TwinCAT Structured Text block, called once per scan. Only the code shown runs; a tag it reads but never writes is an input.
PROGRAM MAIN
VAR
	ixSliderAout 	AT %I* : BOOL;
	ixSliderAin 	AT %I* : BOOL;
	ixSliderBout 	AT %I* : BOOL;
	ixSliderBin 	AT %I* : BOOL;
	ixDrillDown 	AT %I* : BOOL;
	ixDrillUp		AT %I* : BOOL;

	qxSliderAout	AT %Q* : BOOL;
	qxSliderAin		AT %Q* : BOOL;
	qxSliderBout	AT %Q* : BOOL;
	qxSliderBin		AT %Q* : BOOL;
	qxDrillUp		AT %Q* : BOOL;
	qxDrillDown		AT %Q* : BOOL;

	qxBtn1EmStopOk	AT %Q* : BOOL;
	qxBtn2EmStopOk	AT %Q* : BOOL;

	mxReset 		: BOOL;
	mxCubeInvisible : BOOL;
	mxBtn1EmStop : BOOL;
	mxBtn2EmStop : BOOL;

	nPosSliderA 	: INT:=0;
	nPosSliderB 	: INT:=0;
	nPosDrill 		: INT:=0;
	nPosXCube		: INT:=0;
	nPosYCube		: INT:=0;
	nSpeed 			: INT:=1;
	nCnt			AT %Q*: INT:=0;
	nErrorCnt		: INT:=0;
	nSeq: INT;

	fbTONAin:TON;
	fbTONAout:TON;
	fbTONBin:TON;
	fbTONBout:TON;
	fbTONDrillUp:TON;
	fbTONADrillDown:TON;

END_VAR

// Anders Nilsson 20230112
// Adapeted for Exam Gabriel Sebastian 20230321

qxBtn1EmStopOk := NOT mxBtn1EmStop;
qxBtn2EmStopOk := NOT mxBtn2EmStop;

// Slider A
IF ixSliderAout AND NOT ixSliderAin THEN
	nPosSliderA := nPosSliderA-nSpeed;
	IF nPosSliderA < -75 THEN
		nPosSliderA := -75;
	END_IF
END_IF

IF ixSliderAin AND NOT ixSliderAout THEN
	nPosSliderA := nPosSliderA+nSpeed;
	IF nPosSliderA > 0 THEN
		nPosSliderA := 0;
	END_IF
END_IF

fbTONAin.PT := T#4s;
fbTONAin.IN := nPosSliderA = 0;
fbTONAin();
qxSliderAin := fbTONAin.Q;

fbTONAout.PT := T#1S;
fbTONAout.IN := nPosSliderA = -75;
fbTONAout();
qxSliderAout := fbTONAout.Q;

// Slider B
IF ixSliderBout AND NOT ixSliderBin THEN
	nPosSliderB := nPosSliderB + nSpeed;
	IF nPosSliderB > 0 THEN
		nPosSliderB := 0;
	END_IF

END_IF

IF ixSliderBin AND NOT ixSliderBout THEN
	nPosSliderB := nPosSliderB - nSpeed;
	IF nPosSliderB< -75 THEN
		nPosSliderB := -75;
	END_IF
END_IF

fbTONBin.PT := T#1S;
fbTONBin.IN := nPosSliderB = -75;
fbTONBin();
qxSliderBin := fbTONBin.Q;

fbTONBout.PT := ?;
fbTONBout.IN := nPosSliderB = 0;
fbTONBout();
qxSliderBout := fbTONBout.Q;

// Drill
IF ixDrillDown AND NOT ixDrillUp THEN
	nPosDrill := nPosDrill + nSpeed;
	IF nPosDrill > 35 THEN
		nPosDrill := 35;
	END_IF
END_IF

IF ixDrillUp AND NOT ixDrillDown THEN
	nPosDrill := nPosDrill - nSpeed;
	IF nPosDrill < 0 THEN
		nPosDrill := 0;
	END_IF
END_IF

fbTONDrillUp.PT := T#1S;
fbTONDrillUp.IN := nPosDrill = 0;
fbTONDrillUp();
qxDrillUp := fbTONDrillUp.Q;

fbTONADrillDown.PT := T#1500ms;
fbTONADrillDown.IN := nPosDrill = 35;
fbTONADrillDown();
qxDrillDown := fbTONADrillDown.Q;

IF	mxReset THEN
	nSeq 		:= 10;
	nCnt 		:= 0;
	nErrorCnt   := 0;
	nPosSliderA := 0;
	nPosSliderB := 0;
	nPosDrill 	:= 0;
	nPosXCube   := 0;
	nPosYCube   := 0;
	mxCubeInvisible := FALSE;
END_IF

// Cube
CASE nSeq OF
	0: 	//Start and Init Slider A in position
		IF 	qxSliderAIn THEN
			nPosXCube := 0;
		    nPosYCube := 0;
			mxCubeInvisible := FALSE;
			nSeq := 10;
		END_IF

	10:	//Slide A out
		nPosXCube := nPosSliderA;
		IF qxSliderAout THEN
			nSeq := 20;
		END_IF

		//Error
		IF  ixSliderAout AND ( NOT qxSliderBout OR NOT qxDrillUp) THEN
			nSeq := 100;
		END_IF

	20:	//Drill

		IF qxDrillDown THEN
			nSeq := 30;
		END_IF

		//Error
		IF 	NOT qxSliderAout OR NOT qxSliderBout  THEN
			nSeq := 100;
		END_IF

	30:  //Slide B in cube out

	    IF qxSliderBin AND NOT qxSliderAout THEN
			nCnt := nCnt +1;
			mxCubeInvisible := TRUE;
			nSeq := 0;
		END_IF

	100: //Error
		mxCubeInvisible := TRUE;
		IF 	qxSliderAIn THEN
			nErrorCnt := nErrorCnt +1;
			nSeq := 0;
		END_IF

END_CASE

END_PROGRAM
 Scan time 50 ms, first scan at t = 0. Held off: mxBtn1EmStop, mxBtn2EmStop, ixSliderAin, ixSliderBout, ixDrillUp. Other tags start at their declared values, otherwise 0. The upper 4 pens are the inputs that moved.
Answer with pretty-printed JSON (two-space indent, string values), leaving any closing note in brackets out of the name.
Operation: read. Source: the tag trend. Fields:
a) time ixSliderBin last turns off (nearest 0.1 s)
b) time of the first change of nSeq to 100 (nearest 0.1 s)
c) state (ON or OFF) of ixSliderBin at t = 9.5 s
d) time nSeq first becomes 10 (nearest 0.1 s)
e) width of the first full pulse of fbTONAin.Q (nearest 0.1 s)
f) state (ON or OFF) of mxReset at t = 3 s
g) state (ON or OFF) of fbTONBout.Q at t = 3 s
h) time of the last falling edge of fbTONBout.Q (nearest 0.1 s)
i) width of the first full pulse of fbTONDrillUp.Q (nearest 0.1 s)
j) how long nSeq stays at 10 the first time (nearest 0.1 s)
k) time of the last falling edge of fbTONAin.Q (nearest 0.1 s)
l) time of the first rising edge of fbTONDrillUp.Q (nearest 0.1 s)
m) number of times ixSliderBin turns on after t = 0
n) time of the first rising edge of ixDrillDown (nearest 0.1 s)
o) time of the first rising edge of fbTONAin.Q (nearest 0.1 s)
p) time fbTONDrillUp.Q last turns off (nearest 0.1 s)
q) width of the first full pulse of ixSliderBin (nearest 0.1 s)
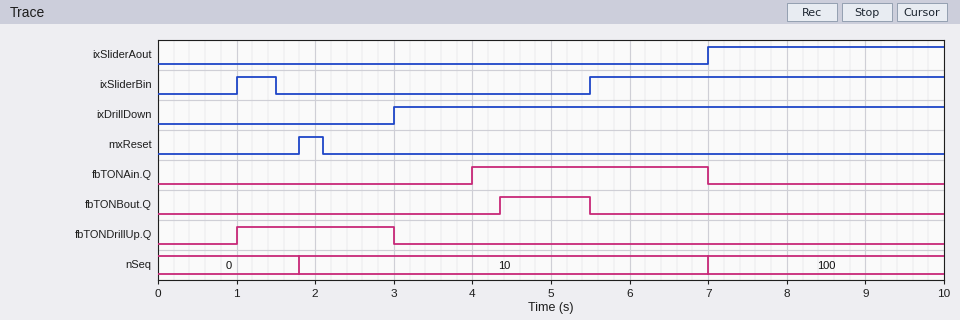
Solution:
{
  "time ixSliderBin last turns off": "1.5 s",
  "time of the first change of nSeq to 100": "7.0 s",
  "state (ON or OFF) of ixSliderBin at t = 9.5 s": "ON",
  "time nSeq first becomes 10": "1.8 s",
  "width of the first full pulse of fbTONAin.Q": "3.0 s",
  "state (ON or OFF) of mxReset at t = 3 s": "OFF",
  "state (ON or OFF) of fbTONBout.Q at t = 3 s": "OFF",
  "time of the last falling edge of fbTONBout.Q": "5.5 s",
  "width of the first full pulse of fbTONDrillUp.Q": "2.0 s",
  "how long nSeq stays at 10 the first time": "5.2 s",
  "time of the last falling edge of fbTONAin.Q": "7.0 s",
  "time of the first rising edge of fbTONDrillUp.Q": "1.0 s",
  "number of times ixSliderBin turns on after t = 0": "2",
  "time of the first rising edge of ixDrillDown": "3.0 s",
  "time of the first rising edge of fbTONAin.Q": "4.0 s",
  "time fbTONDrillUp.Q last turns off": "3.0 s",
  "width of the first full pulse of ixSliderBin": "0.5 s"
}
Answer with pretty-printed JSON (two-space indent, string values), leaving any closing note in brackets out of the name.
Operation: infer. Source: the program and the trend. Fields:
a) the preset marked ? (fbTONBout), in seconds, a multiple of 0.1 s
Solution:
{
  "the preset marked ? (fbTONBout), in seconds, a multiple of 0.1 s": "2.5 s"
}
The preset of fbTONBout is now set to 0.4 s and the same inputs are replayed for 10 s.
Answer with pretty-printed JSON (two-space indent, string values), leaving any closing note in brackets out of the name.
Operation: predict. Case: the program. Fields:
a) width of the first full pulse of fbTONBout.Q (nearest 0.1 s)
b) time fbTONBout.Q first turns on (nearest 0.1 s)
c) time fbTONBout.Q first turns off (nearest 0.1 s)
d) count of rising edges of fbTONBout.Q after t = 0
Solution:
{
  "width of the first full pulse of fbTONBout.Q": "0.6 s",
  "time fbTONBout.Q first turns on": "0.4 s",
  "time fbTONBout.Q first turns off": "1.0 s",
  "count of rising edges of fbTONBout.Q after t = 0": "2"
}
